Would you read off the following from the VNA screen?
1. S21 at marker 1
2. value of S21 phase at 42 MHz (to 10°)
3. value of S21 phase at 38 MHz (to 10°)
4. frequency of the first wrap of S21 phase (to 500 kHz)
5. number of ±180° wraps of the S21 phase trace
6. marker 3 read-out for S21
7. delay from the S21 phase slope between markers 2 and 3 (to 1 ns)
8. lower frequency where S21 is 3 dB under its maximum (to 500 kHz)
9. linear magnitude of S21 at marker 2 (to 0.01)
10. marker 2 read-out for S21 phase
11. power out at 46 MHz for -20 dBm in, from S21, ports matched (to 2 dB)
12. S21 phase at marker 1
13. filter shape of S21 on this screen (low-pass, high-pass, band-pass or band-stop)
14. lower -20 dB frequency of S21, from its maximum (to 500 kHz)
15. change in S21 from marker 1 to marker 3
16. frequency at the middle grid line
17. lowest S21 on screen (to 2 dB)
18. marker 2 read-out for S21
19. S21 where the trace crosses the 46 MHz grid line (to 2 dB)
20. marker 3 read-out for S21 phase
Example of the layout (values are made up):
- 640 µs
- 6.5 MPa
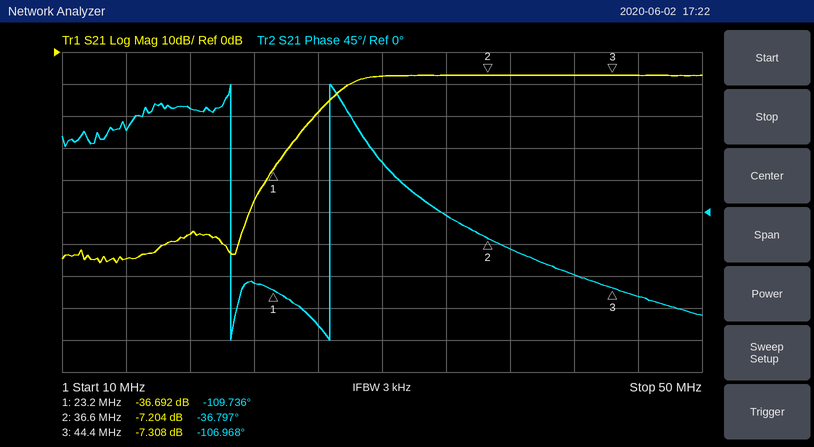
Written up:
- -36.692 dB
- -90°
- -50°
- 20.5 MHz
- 2
- -7.308 dB
- 25 ns
- 28.0 MHz
- 0.44
- -36.797°
- -28 dBm
- -109.736°
- high-pass
- 24.5 MHz
- 29.384 dB
- 30 MHz
- -66 dB
- -7.204 dB
- -8 dB
- -106.968°
